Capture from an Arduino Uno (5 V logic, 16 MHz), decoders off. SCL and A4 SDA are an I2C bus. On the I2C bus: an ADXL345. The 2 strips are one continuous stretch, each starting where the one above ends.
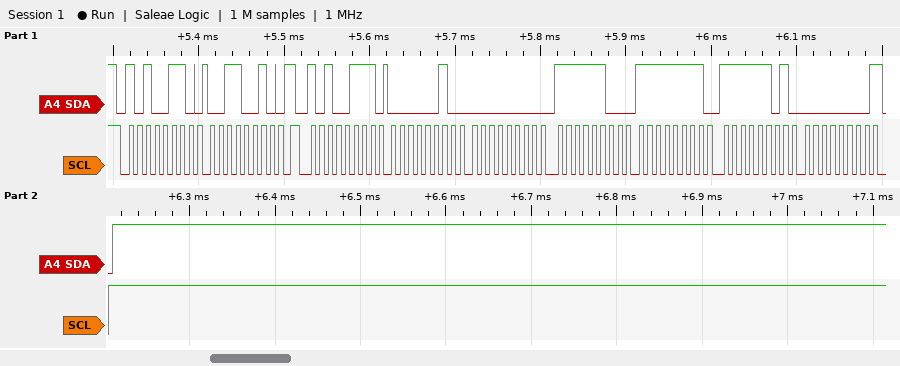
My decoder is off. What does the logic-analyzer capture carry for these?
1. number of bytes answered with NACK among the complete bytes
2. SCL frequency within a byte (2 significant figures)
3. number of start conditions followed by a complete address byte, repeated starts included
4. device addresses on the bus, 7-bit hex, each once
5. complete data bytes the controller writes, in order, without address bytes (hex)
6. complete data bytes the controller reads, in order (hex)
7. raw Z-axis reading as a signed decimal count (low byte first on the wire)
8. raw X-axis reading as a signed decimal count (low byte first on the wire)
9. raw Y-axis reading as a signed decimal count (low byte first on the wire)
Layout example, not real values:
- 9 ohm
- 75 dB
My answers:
- 1
- 100 kHz
- 2
- 0x53
- 32
- 02 00 FC FF FD 00
- 253
- 2
- -4
